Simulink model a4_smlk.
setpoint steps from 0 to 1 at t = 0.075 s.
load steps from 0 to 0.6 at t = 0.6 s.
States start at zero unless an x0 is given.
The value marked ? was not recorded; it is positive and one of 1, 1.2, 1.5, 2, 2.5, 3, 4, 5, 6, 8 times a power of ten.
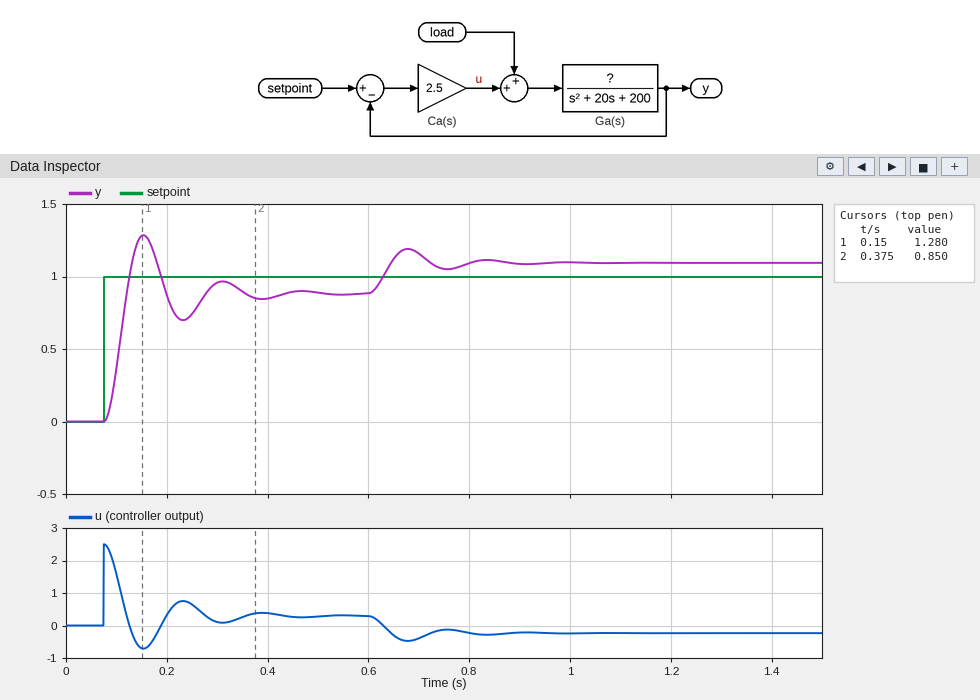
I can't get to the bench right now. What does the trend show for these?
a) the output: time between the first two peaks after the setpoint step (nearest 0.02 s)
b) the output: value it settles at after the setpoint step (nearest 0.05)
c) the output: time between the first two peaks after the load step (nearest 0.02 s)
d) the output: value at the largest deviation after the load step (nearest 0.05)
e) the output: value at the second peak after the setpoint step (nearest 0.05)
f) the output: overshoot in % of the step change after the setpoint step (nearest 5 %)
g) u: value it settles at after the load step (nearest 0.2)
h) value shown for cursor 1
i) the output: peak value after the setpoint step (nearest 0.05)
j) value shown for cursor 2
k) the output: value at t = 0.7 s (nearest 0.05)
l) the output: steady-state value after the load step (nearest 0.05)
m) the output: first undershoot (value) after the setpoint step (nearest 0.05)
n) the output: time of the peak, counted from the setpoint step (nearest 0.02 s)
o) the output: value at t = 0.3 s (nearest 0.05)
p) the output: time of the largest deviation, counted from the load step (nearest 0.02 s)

0.16 s
0.90
0.16 s
1.20
0.95
45 %
-0.2
1.280
1.30
0.850
1.15
1.10
0.70
0.08 s
0.95
0.08 s
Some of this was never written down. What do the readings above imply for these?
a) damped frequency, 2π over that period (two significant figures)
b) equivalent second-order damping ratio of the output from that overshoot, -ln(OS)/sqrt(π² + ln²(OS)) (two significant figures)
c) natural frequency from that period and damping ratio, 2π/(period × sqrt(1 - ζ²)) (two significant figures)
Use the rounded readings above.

39 rad/s
0.25
41 rad/s
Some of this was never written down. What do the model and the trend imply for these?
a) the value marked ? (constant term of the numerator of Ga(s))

600
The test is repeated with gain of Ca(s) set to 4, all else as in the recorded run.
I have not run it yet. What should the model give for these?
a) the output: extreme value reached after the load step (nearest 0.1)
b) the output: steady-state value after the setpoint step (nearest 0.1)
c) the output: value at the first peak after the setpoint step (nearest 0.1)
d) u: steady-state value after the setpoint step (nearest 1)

1.1
0.9
1.4
0
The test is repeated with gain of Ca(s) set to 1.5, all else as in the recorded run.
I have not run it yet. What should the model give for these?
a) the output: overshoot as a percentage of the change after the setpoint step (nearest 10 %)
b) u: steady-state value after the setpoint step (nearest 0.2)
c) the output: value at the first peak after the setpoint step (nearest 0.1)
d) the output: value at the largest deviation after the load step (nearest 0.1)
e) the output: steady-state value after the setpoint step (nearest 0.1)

40 %
0.2
1.1
1.3
0.8
